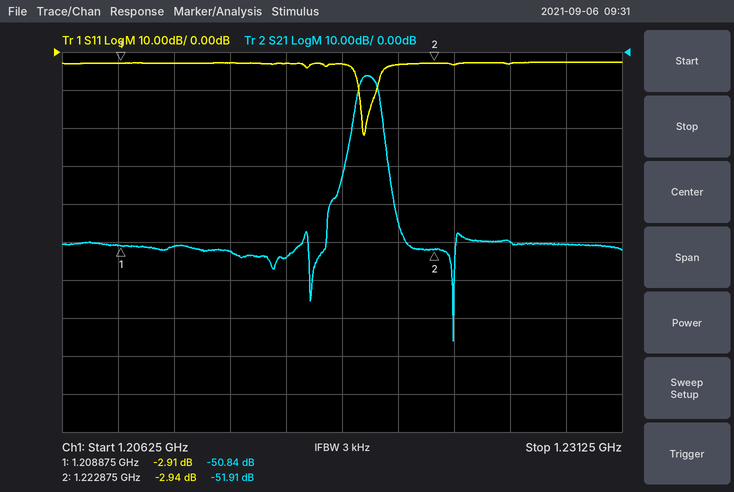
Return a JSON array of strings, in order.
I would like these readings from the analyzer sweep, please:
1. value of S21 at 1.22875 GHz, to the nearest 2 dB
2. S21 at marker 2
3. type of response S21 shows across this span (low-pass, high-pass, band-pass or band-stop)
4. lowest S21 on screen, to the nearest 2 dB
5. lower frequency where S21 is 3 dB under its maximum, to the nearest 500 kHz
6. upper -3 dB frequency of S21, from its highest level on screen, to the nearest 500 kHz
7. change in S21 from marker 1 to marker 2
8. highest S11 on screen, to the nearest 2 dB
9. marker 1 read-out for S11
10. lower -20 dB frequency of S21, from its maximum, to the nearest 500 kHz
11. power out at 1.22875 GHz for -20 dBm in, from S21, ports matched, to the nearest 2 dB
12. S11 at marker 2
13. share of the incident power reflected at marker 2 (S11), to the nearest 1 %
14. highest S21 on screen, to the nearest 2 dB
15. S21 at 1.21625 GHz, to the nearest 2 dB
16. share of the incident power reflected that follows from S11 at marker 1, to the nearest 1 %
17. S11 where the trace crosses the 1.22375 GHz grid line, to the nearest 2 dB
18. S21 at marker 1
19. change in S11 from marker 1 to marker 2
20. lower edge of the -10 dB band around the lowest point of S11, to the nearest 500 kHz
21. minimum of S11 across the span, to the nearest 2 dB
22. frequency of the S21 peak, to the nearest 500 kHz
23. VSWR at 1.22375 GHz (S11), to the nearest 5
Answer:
["-50 dB", "-51.91 dB", "band-pass", "-76 dB", "1.2195 GHz", "1.2205 GHz", "-1.07 dB", "-2 dB", "-2.91 dB", "1.2190 GHz", "-70 dBm", "-2.94 dB", "51 %", "-6 dB", "-54 dB", "51 %", "-4 dB", "-50.84 dB", "-0.03 dB", "1.2195 GHz", "-22 dB", "1.2200 GHz", "5"]
